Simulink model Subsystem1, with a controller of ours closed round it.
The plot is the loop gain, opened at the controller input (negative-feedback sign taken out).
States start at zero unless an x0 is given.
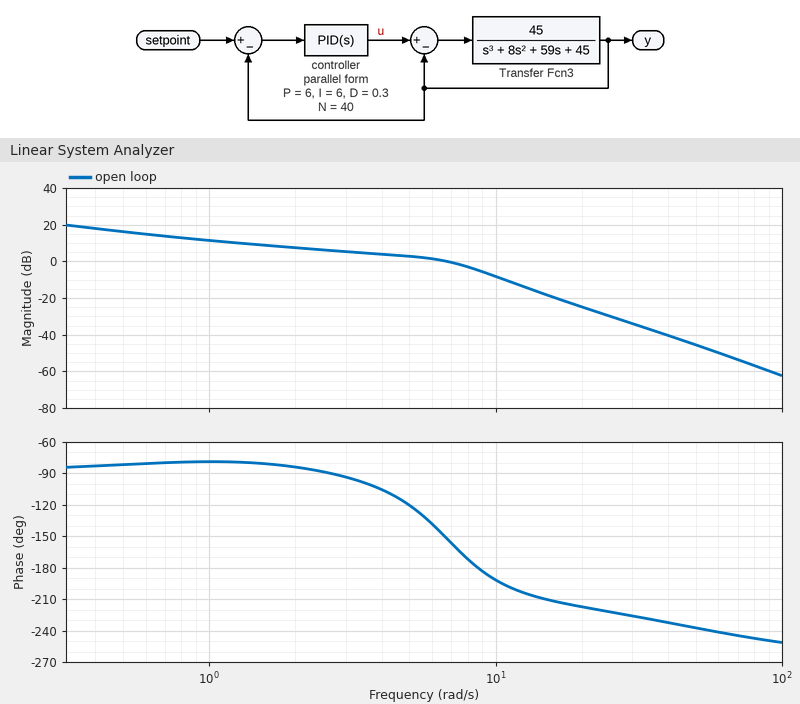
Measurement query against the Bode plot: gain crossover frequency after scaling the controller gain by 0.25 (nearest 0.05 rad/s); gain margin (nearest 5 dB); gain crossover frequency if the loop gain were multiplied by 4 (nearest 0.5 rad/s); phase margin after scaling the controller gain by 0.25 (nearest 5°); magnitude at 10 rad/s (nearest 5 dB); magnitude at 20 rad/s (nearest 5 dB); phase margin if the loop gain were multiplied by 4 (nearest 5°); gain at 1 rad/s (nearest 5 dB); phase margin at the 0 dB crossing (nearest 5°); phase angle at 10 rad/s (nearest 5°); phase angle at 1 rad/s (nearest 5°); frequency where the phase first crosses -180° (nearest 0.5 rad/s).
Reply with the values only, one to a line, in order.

0.90 rad/s
5 dB
11.5 rad/s
100°
-10 dB
-25 dB
-20°
10 dB
30°
-190°
-80°
8.5 rad/s
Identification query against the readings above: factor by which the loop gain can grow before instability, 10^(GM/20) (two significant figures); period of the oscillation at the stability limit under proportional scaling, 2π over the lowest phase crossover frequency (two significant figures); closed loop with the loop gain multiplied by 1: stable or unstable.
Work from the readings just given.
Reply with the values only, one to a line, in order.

1.8
0.74 s
stable
